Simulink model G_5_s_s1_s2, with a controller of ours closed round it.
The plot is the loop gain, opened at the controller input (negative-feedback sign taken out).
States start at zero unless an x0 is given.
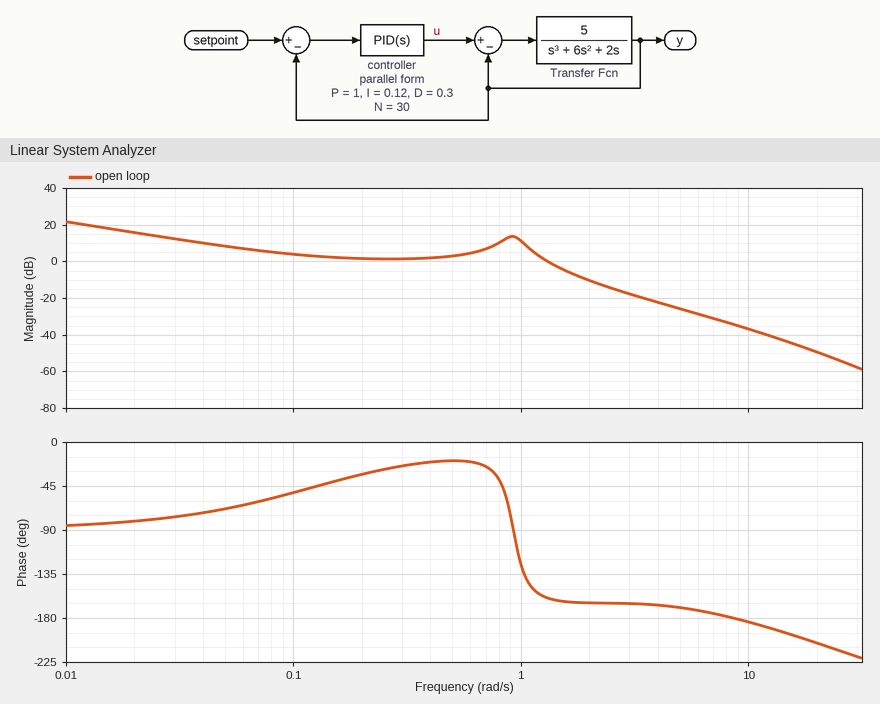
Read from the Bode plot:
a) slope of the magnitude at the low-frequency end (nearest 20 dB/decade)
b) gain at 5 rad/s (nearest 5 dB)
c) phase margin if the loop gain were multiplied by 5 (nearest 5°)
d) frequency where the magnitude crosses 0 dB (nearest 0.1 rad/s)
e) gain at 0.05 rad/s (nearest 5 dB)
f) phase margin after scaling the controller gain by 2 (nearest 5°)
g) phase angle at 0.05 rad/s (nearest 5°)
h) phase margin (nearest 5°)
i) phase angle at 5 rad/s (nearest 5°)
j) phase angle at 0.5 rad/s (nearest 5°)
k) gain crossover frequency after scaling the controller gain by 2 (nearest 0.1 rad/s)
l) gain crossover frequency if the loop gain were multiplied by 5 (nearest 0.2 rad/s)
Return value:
-20 dB/decade
-25 dB
15°
1.3 rad/s
10 dB
15°
-70°
20°
-170°
-20°
1.6 rad/s
2.4 rad/s
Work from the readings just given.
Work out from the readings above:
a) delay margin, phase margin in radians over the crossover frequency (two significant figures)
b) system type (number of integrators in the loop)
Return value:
0.27 s
1
